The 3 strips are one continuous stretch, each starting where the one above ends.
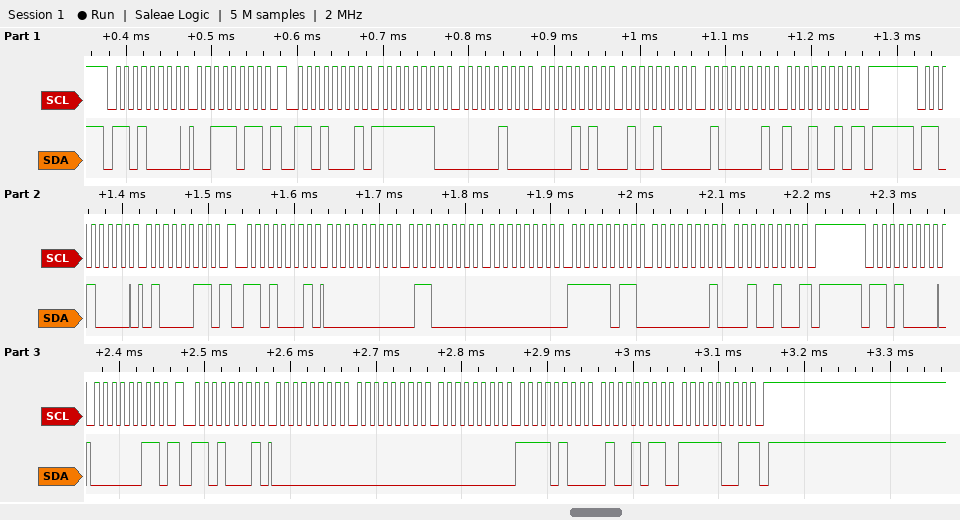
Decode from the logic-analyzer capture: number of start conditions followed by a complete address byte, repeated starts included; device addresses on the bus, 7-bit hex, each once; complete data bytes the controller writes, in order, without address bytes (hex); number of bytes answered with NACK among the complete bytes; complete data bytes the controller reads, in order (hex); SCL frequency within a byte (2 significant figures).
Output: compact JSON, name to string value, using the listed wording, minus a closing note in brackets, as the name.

{"number of start conditions followed by a complete address byte, repeated starts included": "6", "device addresses on the bus, 7-bit hex, each once": "0x68", "complete data bytes the controller writes, in order, without address bytes": "3B 43 03", "number of bytes answered with NACK among the complete bytes": "3", "complete data bytes the controller reads, in order": "FE 04 0A 48 41 92 00 60 00 FB 01 24 00 00 00 F4 4B F9", "SCL frequency within a byte": "100 kHz"}
